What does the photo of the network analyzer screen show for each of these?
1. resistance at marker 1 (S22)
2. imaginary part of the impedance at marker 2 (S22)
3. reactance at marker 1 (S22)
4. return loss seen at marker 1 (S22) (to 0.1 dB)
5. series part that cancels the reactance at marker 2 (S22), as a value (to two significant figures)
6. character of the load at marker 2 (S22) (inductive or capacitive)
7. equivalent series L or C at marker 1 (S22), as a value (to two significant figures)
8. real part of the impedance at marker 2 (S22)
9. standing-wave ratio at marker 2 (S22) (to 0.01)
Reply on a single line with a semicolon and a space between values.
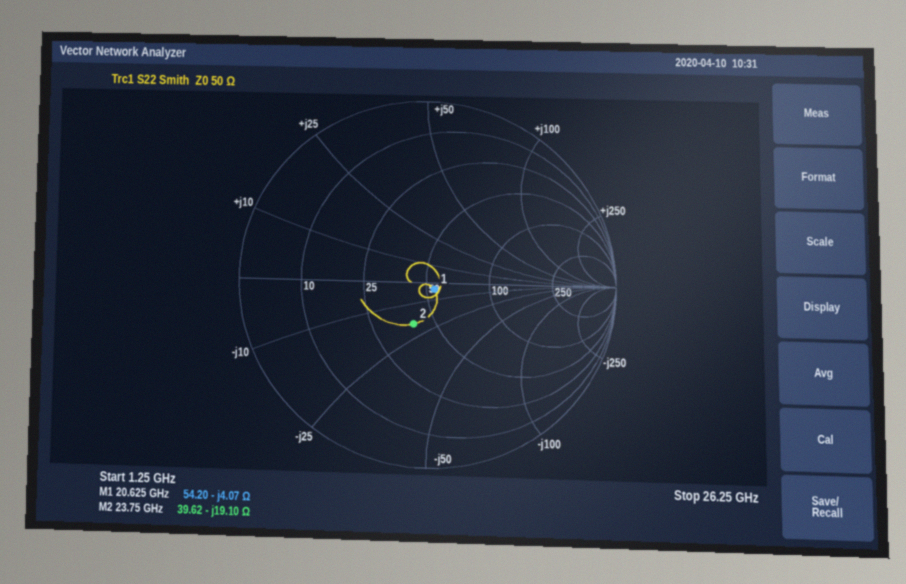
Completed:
54.20 Ω; -19.10 Ω; -4.07 Ω; 25.0 dB; 130 pH; capacitive; 1.9 pF; 39.62 Ω; 1.62
